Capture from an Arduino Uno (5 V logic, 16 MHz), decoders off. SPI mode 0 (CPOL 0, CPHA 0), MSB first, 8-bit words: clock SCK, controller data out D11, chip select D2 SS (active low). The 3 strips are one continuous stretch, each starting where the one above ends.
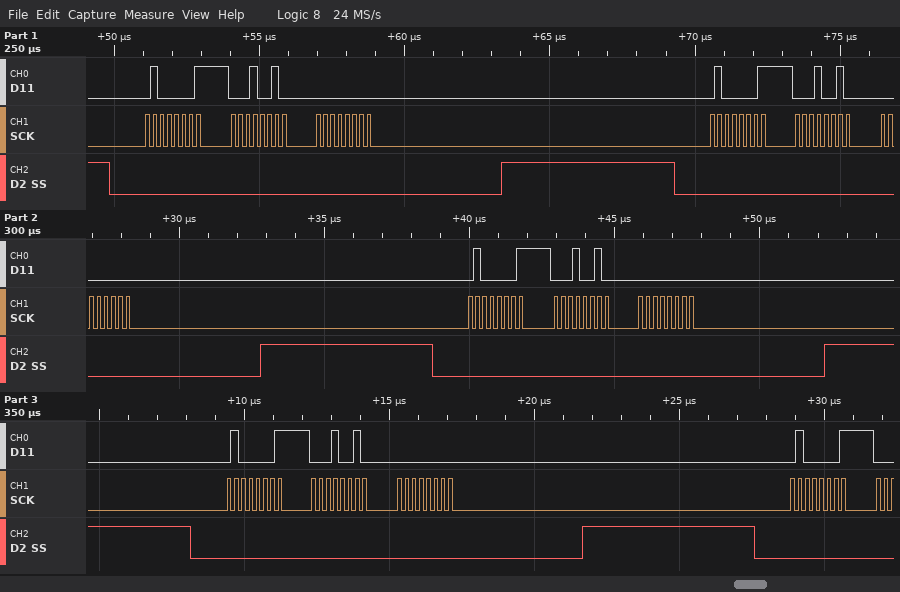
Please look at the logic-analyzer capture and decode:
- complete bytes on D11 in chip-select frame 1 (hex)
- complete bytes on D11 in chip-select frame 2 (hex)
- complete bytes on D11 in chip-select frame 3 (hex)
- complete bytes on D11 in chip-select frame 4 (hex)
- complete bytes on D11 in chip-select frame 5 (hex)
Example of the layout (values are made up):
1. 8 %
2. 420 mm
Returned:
1. 41 12 00
2. 41 12 00
3. 41 12 00
4. 41 12 00
5. 41
